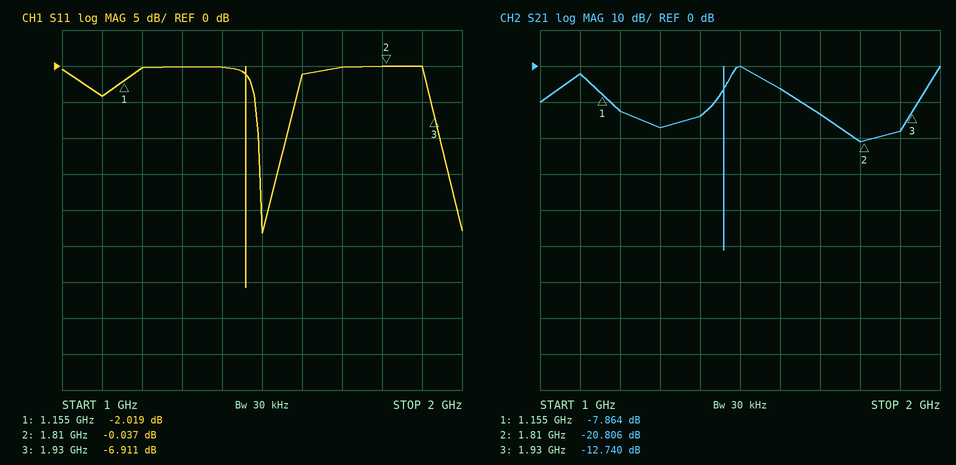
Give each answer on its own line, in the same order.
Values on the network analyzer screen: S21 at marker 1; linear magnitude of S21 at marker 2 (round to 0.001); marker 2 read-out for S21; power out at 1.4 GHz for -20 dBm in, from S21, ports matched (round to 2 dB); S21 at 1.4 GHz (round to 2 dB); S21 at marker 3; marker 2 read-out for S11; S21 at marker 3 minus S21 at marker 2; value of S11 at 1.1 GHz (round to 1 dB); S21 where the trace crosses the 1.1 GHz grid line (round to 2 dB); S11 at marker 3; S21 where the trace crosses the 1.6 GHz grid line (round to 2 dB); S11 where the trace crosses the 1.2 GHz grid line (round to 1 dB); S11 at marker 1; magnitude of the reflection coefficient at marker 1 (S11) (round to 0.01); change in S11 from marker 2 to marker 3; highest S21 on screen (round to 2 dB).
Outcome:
-7.864 dB
0.091
-20.806 dB
-34 dBm
-14 dB
-12.740 dB
-0.037 dB
8.066 dB
-4 dB
-2 dB
-6.911 dB
-6 dB
0 dB
-2.019 dB
0.79
-6.874 dB
0 dB
